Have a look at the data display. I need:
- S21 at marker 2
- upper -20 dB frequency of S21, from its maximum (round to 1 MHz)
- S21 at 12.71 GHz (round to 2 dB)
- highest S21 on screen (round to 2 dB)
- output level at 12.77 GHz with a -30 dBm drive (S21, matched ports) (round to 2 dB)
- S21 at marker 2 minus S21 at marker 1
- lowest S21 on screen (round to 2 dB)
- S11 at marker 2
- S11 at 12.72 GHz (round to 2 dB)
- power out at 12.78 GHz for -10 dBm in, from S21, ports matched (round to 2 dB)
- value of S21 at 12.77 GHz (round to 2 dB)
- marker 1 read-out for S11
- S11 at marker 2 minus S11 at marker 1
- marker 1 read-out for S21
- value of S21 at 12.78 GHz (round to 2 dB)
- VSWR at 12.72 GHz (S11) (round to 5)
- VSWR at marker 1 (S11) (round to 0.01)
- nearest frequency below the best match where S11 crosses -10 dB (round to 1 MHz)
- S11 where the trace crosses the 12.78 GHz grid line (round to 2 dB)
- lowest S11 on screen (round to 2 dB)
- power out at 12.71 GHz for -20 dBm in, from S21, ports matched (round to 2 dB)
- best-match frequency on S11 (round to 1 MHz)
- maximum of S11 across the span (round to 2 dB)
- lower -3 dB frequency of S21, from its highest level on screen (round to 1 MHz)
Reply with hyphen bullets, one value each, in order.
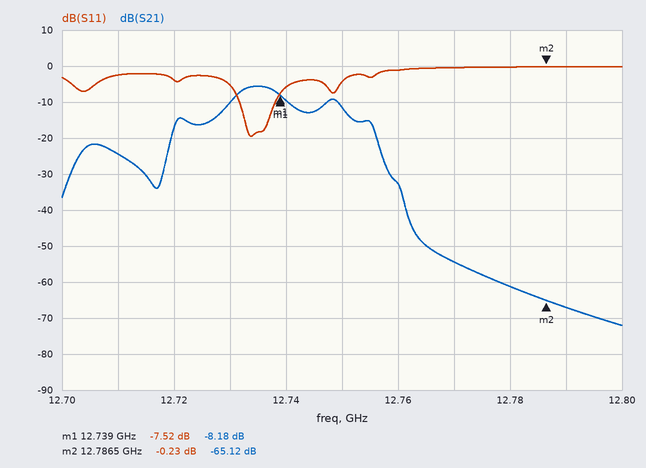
- -65.12 dB
- 12.757 GHz
- -24 dB
- -6 dB
- -84 dBm
- -56.94 dB
- -72 dB
- -0.23 dB
- -4 dB
- -72 dBm
- -54 dB
- -7.52 dB
- 7.29 dB
- -8.18 dB
- -62 dB
- 5
- 2.45
- 12.732 GHz
- 0 dB
- -20 dB
- -44 dBm
- 12.734 GHz
- 0 dB
- 12.731 GHz
